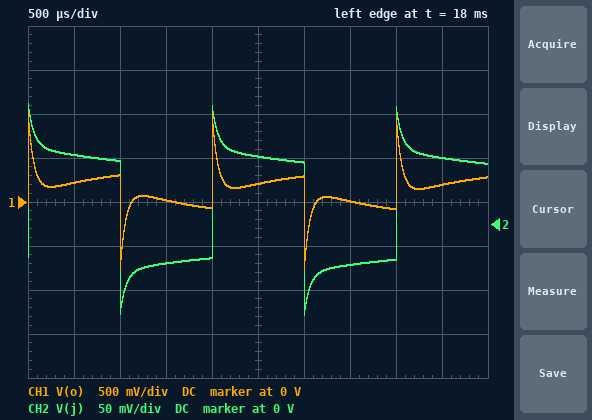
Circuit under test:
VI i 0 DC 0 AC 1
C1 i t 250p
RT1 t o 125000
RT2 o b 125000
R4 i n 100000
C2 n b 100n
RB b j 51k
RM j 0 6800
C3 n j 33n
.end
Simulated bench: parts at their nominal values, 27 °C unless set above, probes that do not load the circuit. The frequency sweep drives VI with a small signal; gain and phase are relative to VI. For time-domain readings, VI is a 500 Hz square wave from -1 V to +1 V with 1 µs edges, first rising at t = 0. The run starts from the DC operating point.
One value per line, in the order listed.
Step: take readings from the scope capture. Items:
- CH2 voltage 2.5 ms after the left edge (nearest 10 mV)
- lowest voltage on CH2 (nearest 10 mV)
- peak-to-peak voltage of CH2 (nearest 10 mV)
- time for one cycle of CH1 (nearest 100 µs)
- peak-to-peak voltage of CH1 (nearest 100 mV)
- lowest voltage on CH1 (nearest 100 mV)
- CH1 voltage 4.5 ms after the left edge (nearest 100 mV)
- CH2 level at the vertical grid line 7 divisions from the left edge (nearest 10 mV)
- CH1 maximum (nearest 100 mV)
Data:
80 mV
-100 mV
240 mV
2.0 ms
1.8 V
-800 mV
200 mV
-50 mV
1.0 V
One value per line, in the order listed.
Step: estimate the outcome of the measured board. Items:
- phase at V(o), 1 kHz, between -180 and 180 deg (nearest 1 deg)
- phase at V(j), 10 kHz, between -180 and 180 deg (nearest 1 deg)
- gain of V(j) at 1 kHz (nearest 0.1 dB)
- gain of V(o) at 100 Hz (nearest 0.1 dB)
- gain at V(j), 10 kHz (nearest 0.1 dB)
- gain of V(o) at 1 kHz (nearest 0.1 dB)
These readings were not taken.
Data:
42 deg
4 deg
-23.5 dB
-11.2 dB
-21.3 dB
-14.7 dB
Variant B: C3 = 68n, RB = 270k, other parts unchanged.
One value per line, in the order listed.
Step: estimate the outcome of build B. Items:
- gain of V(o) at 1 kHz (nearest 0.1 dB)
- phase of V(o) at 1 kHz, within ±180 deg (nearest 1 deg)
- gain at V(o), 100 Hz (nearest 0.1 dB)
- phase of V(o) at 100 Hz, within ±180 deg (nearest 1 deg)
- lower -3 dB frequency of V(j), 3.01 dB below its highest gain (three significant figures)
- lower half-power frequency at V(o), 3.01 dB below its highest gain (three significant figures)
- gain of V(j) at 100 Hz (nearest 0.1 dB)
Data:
-14.2 dB
48 deg
-13.5 dB
-51 deg
111 Hz
3.24 Hz
-24.3 dB
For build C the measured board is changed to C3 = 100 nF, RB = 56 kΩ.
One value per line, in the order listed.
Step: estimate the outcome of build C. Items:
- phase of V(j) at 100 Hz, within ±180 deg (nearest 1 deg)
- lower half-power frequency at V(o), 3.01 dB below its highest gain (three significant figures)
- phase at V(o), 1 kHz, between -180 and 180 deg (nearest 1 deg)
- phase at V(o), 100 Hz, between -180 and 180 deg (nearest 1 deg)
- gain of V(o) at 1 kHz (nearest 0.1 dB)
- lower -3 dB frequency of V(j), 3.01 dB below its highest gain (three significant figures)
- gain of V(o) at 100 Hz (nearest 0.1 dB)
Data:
8 deg
2.50 kHz
49 deg
-28 deg
-13.9 dB
109 Hz
-16.2 dB
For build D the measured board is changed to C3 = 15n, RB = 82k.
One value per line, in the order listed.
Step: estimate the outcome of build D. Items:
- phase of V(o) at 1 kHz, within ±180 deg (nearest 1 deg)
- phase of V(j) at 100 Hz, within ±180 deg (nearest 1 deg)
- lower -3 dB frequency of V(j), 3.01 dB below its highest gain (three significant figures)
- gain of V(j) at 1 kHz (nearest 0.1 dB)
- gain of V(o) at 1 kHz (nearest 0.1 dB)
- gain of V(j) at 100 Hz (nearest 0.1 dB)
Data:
28 deg
16 deg
595 Hz
-23.7 dB
-15.5 dB
-27.2 dB
